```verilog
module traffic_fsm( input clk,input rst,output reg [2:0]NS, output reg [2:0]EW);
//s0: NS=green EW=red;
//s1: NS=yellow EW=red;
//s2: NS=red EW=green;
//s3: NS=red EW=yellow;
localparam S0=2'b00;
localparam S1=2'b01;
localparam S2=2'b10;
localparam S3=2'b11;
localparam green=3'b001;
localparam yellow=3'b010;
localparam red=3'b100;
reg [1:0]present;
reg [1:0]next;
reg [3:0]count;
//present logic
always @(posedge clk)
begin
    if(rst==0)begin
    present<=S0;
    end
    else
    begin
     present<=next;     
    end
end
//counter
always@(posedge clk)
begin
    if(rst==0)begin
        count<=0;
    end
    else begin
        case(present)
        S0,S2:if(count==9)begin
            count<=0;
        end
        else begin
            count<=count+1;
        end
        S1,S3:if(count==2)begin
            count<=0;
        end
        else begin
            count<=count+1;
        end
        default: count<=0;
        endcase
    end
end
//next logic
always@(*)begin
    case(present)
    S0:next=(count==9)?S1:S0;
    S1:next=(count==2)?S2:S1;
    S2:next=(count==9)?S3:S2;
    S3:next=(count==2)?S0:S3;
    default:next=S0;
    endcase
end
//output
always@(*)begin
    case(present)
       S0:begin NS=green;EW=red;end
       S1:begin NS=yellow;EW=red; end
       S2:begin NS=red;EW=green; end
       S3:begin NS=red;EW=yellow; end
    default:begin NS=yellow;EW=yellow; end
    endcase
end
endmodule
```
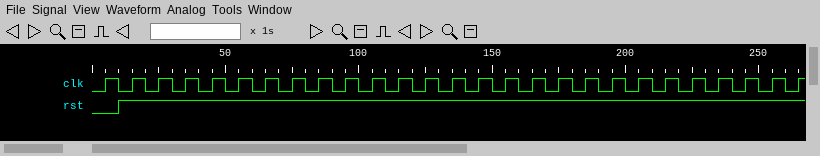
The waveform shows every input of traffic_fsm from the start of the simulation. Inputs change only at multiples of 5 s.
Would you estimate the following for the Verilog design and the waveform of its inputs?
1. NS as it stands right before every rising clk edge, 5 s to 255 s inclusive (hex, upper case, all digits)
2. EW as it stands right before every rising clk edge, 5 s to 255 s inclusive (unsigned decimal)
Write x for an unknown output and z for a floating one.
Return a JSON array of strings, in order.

["x, 1, 1, 1, 1, 1, 1, 1, 1, 1, 1, 2, 2, 2, 4, 4, 4, 4, 4, 4, 4, 4, 4, 4, 4, 4", "x, 4, 4, 4, 4, 4, 4, 4, 4, 4, 4, 4, 4, 4, 1, 1, 1, 1, 1, 1, 1, 1, 1, 1, 2, 2"]
